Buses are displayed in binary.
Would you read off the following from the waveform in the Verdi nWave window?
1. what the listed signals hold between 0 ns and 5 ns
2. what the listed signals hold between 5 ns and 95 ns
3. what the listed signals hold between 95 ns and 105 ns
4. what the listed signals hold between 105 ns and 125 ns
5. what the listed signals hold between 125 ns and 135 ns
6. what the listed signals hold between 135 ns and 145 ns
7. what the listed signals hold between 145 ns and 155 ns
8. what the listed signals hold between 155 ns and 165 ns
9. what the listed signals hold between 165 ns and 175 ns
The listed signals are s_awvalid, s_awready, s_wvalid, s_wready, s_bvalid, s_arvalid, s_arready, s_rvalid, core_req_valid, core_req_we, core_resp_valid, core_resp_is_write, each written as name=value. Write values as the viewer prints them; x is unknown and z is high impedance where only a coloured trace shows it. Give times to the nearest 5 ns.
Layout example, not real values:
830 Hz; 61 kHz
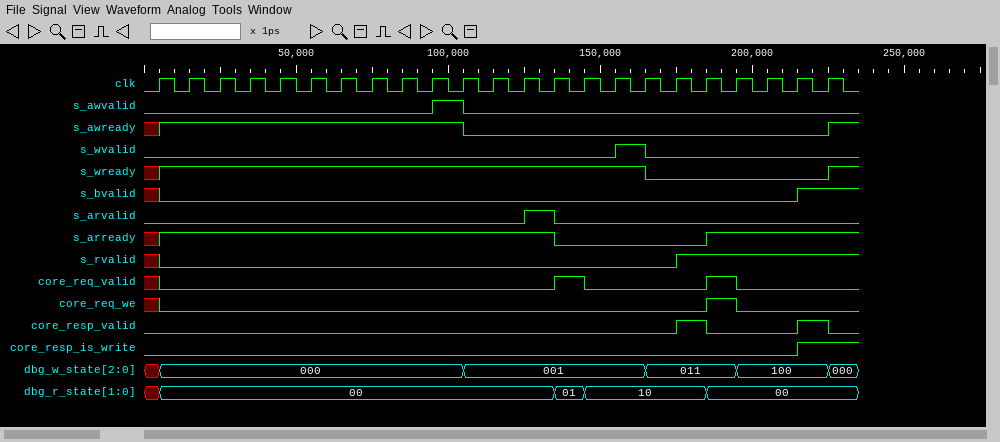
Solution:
s_awvalid=0, s_awready=x, s_wvalid=0, s_wready=x, s_bvalid=x, s_arvalid=0, s_arready=x, s_rvalid=x, core_req_valid=x, core_req_we=x, core_resp_valid=0, core_resp_is_write=0; s_awvalid=0, s_awready=1, s_wvalid=0, s_wready=1, s_bvalid=0, s_arvalid=0, s_arready=1, s_rvalid=0, core_req_valid=0, core_req_we=0, core_resp_valid=0, core_resp_is_write=0; s_awvalid=1, s_awready=1, s_wvalid=0, s_wready=1, s_bvalid=0, s_arvalid=0, s_arready=1, s_rvalid=0, core_req_valid=0, core_req_we=0, core_resp_valid=0, core_resp_is_write=0; s_awvalid=0, s_awready=0, s_wvalid=0, s_wready=1, s_bvalid=0, s_arvalid=0, s_arready=1, s_rvalid=0, core_req_valid=0, core_req_we=0, core_resp_valid=0, core_resp_is_write=0; s_awvalid=0, s_awready=0, s_wvalid=0, s_wready=1, s_bvalid=0, s_arvalid=1, s_arready=1, s_rvalid=0, core_req_valid=0, core_req_we=0, core_resp_valid=0, core_resp_is_write=0; s_awvalid=0, s_awready=0, s_wvalid=0, s_wready=1, s_bvalid=0, s_arvalid=0, s_arready=0, s_rvalid=0, core_req_valid=1, core_req_we=0, core_resp_valid=0, core_resp_is_write=0; s_awvalid=0, s_awready=0, s_wvalid=0, s_wready=1, s_bvalid=0, s_arvalid=0, s_arready=0, s_rvalid=0, core_req_valid=0, core_req_we=0, core_resp_valid=0, core_resp_is_write=0; s_awvalid=0, s_awready=0, s_wvalid=1, s_wready=1, s_bvalid=0, s_arvalid=0, s_arready=0, s_rvalid=0, core_req_valid=0, core_req_we=0, core_resp_valid=0, core_resp_is_write=0; s_awvalid=0, s_awready=0, s_wvalid=0, s_wready=0, s_bvalid=0, s_arvalid=0, s_arready=0, s_rvalid=0, core_req_valid=0, core_req_we=0, core_resp_valid=0, core_resp_is_write=0
